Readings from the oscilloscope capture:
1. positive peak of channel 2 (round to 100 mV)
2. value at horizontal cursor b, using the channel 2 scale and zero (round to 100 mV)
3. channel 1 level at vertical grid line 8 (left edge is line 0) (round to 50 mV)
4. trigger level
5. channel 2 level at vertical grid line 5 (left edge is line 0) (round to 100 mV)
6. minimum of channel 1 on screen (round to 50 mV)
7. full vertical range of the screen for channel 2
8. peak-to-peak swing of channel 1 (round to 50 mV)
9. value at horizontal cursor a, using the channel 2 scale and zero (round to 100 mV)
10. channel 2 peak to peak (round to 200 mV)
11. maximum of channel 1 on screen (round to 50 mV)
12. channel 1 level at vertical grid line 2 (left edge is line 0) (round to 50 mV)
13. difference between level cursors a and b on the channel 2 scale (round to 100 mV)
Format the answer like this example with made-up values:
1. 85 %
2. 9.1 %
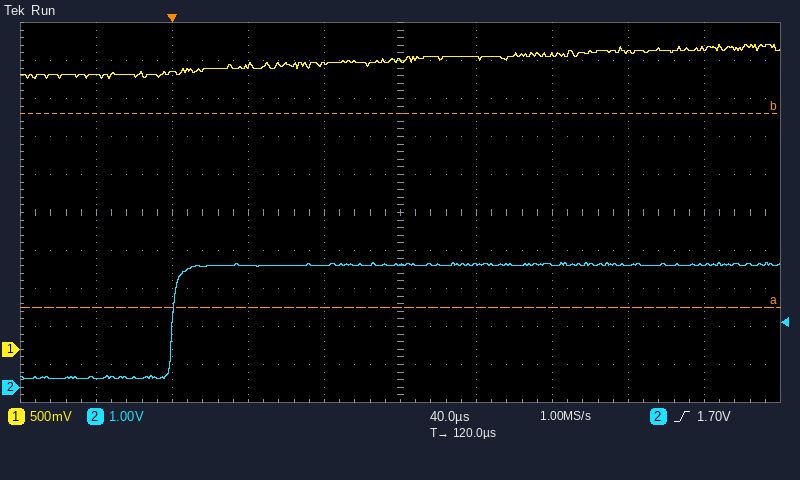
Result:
1. 3.3 V
2. 7.2 V
3. 3.90 V
4. 1.70 V
5. 3.2 V
6. 3.55 V
7. 10 V
8. 450 mV
9. 2.1 V
10. 3.0 V
11. 4.00 V
12. 3.65 V
13. 5.1 V
